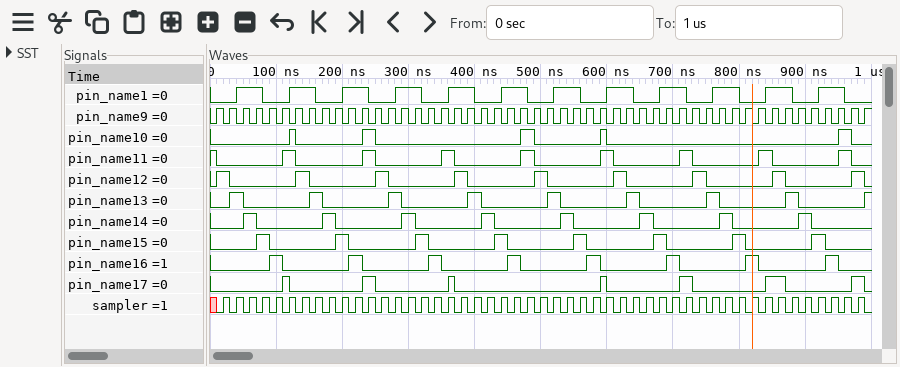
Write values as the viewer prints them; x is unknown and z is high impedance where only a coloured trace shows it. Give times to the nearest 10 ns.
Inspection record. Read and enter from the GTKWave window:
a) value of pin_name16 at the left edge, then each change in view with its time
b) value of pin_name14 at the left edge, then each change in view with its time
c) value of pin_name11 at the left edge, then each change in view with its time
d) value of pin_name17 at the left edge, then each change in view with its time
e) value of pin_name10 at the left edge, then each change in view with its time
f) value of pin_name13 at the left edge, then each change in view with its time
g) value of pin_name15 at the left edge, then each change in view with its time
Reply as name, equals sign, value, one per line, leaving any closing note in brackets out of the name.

value of pin_name16 at the left edge, then each change in view with its time = 0, 1 at 90 ns, 0 at 110 ns, 1 at 210 ns, 0 at 230 ns, 1 at 330 ns, 0 at 350 ns, 1 at 450 ns, 0 at 470 ns, 1 at 570 ns, 0 at 590 ns, 1 at 690 ns, 0 at 710 ns, 1 at 810 ns, 0 at 830 ns, 1 at 930 ns, 0 at 950 ns
value of pin_name14 at the left edge, then each change in view with its time = 0, 1 at 50 ns, 0 at 70 ns, 1 at 170 ns, 0 at 190 ns, 1 at 290 ns, 0 at 310 ns, 1 at 410 ns, 0 at 430 ns, 1 at 530 ns, 0 at 550 ns, 1 at 650 ns, 0 at 670 ns, 1 at 770 ns, 0 at 790 ns, 1 at 890 ns, 0 at 910 ns
value of pin_name11 at the left edge, then each change in view with its time = 1, 0 at 10 ns, 1 at 110 ns, 0 at 130 ns, 1 at 230 ns, 0 at 250 ns, 1 at 350 ns, 0 at 370 ns, 1 at 470 ns, 0 at 490 ns, 1 at 590 ns, 0 at 610 ns, 1 at 710 ns, 0 at 730 ns, 1 at 830 ns, 0 at 850 ns, 1 at 950 ns, 0 at 970 ns
value of pin_name17 at the left edge, then each change in view with its time = 0, 1 at 110 ns, 0 at 120 ns, 1 at 230 ns, 0 at 250 ns, 1 at 360 ns, 0 at 370 ns, 1 at 590 ns, 0 at 600 ns, 1 at 710 ns, 0 at 730 ns, 1 at 840 ns, 0 at 870 ns, 1 at 970 ns, 0 at 990 ns
value of pin_name10 at the left edge, then each change in view with its time = 0, 1 at 120 ns, 0 at 130 ns, 1 at 230 ns, 0 at 250 ns, 1 at 470 ns, 0 at 490 ns, 1 at 590 ns, 0 at 600 ns, 1 at 950 ns, 0 at 970 ns
value of pin_name13 at the left edge, then each change in view with its time = 0, 1 at 30 ns, 0 at 50 ns, 1 at 150 ns, 0 at 170 ns, 1 at 270 ns, 0 at 290 ns, 1 at 390 ns, 0 at 410 ns, 1 at 510 ns, 0 at 530 ns, 1 at 630 ns, 0 at 650 ns, 1 at 750 ns, 0 at 770 ns, 1 at 870 ns, 0 at 890 ns, 1 at 990 ns
value of pin_name15 at the left edge, then each change in view with its time = 0, 1 at 70 ns, 0 at 90 ns, 1 at 190 ns, 0 at 210 ns, 1 at 310 ns, 0 at 330 ns, 1 at 430 ns, 0 at 450 ns, 1 at 550 ns, 0 at 570 ns, 1 at 670 ns, 0 at 690 ns, 1 at 790 ns, 0 at 810 ns, 1 at 910 ns, 0 at 930 ns
